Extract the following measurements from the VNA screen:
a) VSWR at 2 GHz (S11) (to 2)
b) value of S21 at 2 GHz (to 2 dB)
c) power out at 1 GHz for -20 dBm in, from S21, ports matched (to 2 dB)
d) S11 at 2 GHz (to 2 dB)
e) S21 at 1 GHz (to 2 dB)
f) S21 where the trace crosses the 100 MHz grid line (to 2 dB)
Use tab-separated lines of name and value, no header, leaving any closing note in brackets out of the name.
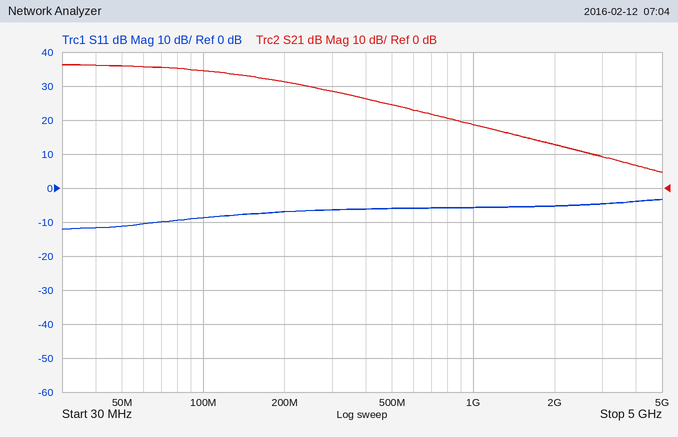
VSWR at 2 GHz (S11)	4
value of S21 at 2 GHz	12 dB
power out at 1 GHz for -20 dBm in, from S21, ports matched	-2 dBm
S11 at 2 GHz	-6 dB
S21 at 1 GHz	18 dB
S21 where the trace crosses the 100 MHz grid line	34 dB
